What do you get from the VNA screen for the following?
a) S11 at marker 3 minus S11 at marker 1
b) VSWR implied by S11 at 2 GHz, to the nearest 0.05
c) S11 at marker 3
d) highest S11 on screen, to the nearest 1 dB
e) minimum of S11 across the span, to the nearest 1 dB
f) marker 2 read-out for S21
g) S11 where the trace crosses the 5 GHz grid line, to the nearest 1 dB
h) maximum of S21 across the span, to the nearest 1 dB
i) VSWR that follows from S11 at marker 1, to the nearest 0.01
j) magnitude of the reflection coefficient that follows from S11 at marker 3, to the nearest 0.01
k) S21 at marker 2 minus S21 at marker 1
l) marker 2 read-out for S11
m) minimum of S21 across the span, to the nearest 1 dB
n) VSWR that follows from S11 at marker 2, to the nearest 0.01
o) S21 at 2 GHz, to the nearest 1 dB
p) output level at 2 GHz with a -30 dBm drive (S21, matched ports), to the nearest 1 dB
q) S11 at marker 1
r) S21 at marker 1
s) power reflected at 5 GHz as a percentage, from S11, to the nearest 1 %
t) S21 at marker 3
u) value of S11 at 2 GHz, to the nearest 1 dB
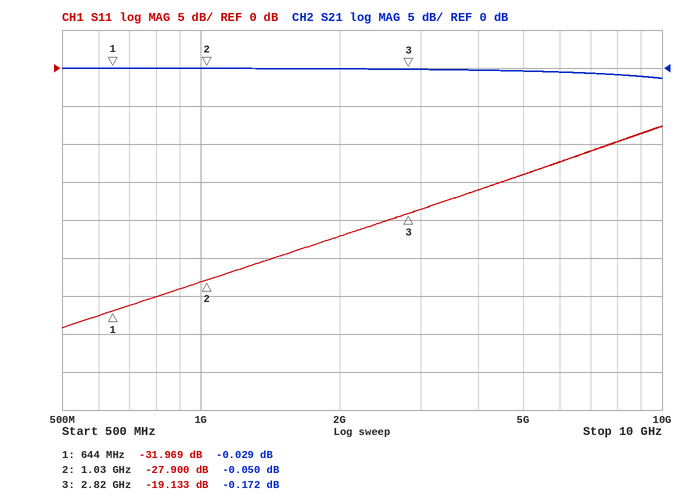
12.836 dB
1.15
-19.133 dB
-8 dB
-34 dB
-0.050 dB
-14 dB
0 dB
1.05
0.11
-0.021 dB
-27.900 dB
-1 dB
1.08
0 dB
-30 dBm
-31.969 dB
-0.029 dB
4 %
-0.172 dB
-22 dB
